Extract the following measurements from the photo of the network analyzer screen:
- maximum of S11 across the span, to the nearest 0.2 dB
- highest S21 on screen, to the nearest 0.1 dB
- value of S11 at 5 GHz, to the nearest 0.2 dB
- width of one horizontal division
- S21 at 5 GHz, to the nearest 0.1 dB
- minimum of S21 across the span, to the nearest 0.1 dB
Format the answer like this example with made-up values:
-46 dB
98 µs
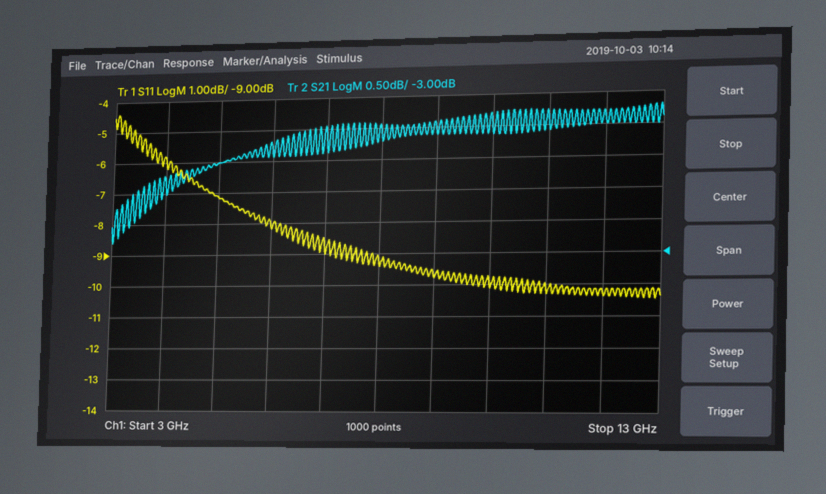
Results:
-4.4 dB
-0.7 dB
-7.2 dB
1 GHz
-1.5 dB
-2.8 dB
